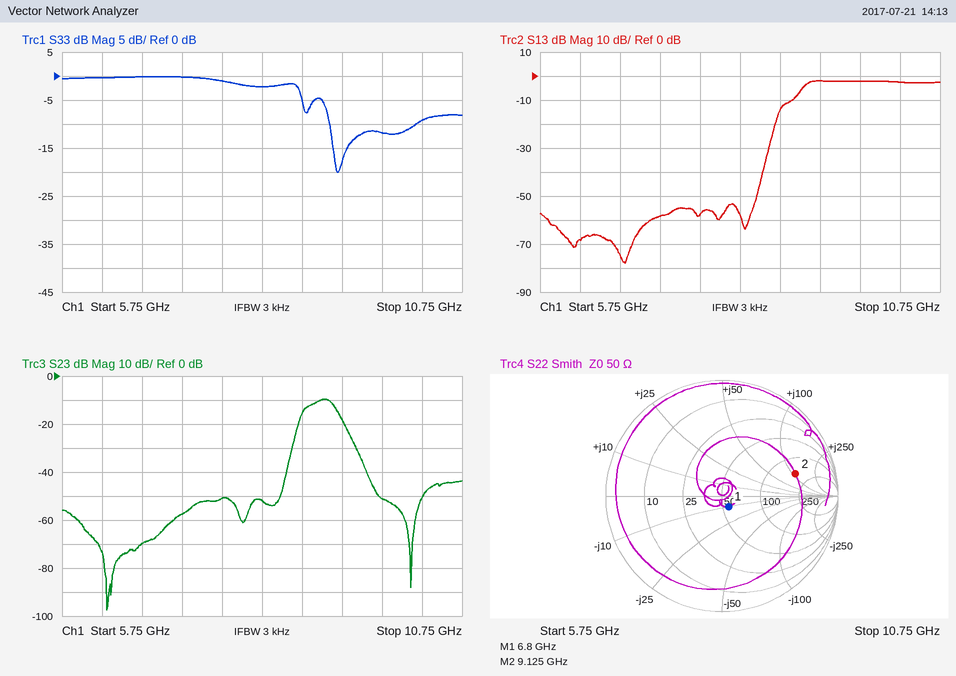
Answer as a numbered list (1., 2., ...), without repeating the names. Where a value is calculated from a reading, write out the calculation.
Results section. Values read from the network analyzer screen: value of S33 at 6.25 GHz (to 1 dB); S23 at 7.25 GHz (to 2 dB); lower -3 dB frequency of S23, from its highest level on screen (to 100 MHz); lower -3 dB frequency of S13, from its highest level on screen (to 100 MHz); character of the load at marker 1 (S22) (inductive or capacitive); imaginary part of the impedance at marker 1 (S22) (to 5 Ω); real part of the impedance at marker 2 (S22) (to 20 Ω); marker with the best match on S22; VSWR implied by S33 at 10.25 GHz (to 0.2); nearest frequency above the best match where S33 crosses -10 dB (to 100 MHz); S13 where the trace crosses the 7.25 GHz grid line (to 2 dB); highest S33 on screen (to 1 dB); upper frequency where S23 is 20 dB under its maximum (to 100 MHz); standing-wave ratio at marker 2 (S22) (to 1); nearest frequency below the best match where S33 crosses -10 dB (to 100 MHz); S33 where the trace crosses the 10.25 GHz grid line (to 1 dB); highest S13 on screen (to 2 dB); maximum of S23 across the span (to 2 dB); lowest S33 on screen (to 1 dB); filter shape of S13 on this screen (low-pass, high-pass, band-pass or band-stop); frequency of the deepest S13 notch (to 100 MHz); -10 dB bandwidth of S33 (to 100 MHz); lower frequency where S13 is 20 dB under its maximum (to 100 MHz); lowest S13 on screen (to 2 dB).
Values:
1. 0 dB
2. -58 dB
3. 8.8 GHz
4. 9.0 GHz
5. capacitive
6. -10 Ω
7. 160 Ω
8. marker 1
9. |Γ| = 10^(-9/20) = 0.3548; VSWR = (1 + 0.3548)/(1 − 0.3548) ≈ 2.10, so 2.0 to the nearest 0.2
10. 10.2 GHz
11. -58 dB
12. 0 dB
13. 9.4 GHz
14. 5
15. 9.1 GHz
16. -9 dB
17. -2 dB
18. -10 dB
19. -20 dB
20. high-pass
21. 6.8 GHz
22. 10.2 GHz − 9.1 GHz = 1.1 GHz
23. 8.7 GHz
24. -78 dB
